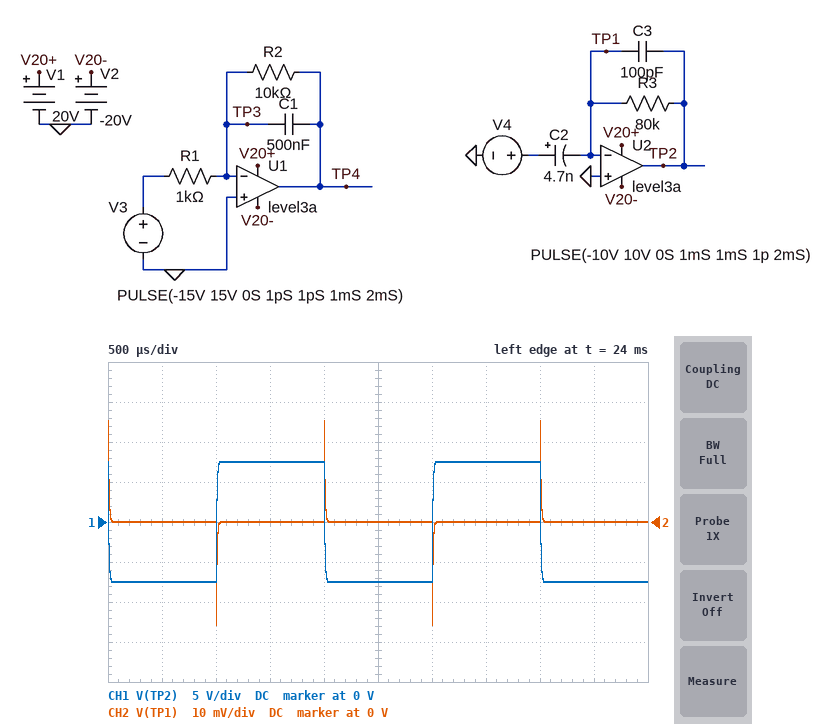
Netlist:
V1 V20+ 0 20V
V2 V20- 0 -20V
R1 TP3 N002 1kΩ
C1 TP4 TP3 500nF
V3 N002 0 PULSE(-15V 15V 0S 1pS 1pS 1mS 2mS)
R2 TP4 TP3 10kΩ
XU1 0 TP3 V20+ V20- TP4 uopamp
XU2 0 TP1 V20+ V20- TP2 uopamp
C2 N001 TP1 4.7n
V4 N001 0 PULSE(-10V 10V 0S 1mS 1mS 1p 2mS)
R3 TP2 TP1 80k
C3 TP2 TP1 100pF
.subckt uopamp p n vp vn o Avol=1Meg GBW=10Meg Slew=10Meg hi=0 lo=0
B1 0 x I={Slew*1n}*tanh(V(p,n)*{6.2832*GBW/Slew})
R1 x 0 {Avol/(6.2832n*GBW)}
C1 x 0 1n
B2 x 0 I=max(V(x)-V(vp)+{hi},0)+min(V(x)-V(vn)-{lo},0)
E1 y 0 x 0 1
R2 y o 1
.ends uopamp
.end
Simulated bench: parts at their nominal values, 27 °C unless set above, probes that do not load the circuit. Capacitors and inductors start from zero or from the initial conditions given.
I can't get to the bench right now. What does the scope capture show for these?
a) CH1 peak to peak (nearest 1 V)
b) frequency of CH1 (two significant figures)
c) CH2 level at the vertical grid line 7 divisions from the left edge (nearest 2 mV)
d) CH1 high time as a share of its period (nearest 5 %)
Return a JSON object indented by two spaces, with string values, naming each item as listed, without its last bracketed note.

{
  "CH1 peak to peak": "15 V",
  "frequency of CH1": "500 Hz",
  "CH2 level at the vertical grid line 7 divisions from the left edge": "0 V",
  "CH1 high time as a share of its period": "50 %"
}
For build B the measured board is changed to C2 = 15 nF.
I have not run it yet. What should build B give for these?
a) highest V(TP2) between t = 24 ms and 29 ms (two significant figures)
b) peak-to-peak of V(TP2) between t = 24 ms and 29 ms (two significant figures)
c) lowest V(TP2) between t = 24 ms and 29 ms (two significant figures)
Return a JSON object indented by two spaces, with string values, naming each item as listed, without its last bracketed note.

{
  "highest V(TP2) between t = 24 ms and 29 ms": "20 V",
  "peak-to-peak of V(TP2) between t = 24 ms and 29 ms": "40 V",
  "lowest V(TP2) between t = 24 ms and 29 ms": "-20 V"
}
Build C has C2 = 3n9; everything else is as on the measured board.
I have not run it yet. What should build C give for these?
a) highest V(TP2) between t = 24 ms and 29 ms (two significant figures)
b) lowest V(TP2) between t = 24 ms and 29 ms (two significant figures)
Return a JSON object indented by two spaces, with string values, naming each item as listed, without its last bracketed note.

{
  "highest V(TP2) between t = 24 ms and 29 ms": "6.2 V",
  "lowest V(TP2) between t = 24 ms and 29 ms": "-6.2 V"
}
